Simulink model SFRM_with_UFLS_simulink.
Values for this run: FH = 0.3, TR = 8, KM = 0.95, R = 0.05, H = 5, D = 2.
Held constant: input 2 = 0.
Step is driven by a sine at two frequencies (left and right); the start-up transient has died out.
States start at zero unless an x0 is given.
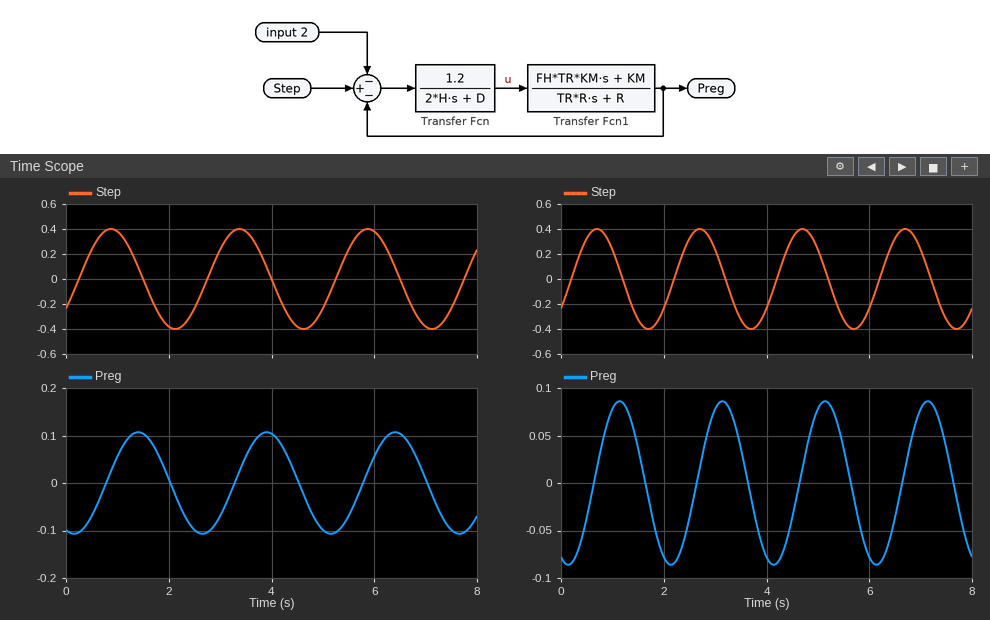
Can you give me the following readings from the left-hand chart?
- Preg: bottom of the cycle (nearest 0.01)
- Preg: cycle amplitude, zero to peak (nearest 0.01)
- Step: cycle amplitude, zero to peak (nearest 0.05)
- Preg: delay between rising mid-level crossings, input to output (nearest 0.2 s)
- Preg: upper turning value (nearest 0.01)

-0.11
0.11
0.40
0.6 s
0.11
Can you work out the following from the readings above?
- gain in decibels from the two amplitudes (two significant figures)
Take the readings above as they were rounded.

-11 dB
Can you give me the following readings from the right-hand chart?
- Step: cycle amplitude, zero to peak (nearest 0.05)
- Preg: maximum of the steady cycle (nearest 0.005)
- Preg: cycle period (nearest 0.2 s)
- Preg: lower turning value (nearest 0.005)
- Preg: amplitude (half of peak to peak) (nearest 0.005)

0.40
0.085
2.0 s
-0.085
0.085
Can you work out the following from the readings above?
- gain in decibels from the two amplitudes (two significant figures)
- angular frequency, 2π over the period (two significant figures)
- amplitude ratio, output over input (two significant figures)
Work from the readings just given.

-13 dB
3.1 rad/s
0.21
